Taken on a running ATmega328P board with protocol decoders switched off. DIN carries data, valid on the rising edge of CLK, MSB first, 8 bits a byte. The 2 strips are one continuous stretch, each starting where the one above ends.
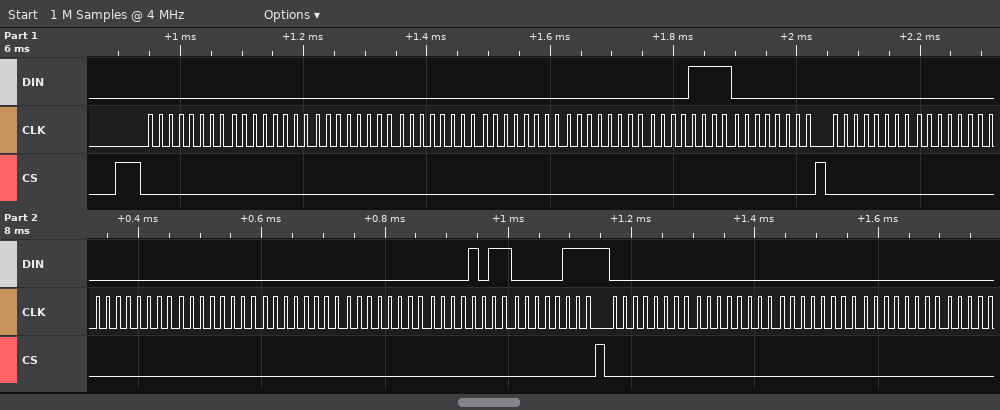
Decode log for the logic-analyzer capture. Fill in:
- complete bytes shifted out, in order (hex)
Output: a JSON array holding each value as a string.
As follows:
["00 00 00 00 00 00 0F 00 00 00 00 00 00 00 0B 07 00 00 00 00"]
